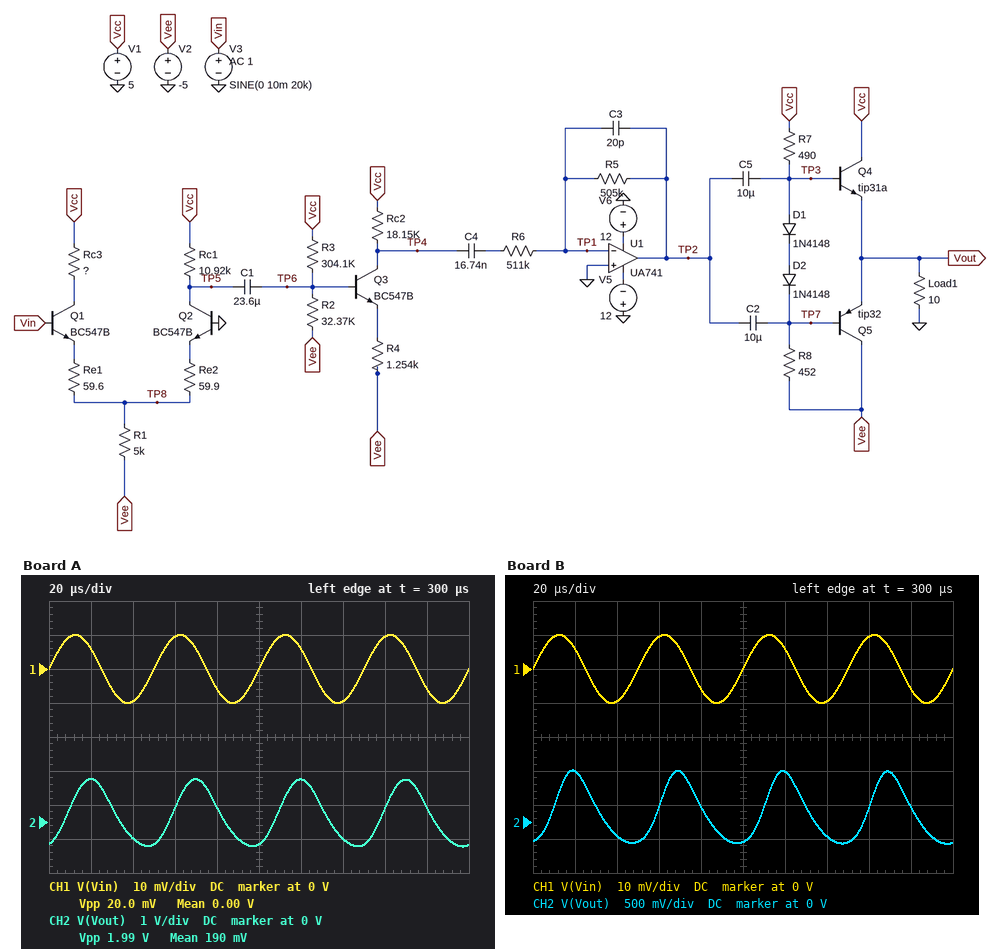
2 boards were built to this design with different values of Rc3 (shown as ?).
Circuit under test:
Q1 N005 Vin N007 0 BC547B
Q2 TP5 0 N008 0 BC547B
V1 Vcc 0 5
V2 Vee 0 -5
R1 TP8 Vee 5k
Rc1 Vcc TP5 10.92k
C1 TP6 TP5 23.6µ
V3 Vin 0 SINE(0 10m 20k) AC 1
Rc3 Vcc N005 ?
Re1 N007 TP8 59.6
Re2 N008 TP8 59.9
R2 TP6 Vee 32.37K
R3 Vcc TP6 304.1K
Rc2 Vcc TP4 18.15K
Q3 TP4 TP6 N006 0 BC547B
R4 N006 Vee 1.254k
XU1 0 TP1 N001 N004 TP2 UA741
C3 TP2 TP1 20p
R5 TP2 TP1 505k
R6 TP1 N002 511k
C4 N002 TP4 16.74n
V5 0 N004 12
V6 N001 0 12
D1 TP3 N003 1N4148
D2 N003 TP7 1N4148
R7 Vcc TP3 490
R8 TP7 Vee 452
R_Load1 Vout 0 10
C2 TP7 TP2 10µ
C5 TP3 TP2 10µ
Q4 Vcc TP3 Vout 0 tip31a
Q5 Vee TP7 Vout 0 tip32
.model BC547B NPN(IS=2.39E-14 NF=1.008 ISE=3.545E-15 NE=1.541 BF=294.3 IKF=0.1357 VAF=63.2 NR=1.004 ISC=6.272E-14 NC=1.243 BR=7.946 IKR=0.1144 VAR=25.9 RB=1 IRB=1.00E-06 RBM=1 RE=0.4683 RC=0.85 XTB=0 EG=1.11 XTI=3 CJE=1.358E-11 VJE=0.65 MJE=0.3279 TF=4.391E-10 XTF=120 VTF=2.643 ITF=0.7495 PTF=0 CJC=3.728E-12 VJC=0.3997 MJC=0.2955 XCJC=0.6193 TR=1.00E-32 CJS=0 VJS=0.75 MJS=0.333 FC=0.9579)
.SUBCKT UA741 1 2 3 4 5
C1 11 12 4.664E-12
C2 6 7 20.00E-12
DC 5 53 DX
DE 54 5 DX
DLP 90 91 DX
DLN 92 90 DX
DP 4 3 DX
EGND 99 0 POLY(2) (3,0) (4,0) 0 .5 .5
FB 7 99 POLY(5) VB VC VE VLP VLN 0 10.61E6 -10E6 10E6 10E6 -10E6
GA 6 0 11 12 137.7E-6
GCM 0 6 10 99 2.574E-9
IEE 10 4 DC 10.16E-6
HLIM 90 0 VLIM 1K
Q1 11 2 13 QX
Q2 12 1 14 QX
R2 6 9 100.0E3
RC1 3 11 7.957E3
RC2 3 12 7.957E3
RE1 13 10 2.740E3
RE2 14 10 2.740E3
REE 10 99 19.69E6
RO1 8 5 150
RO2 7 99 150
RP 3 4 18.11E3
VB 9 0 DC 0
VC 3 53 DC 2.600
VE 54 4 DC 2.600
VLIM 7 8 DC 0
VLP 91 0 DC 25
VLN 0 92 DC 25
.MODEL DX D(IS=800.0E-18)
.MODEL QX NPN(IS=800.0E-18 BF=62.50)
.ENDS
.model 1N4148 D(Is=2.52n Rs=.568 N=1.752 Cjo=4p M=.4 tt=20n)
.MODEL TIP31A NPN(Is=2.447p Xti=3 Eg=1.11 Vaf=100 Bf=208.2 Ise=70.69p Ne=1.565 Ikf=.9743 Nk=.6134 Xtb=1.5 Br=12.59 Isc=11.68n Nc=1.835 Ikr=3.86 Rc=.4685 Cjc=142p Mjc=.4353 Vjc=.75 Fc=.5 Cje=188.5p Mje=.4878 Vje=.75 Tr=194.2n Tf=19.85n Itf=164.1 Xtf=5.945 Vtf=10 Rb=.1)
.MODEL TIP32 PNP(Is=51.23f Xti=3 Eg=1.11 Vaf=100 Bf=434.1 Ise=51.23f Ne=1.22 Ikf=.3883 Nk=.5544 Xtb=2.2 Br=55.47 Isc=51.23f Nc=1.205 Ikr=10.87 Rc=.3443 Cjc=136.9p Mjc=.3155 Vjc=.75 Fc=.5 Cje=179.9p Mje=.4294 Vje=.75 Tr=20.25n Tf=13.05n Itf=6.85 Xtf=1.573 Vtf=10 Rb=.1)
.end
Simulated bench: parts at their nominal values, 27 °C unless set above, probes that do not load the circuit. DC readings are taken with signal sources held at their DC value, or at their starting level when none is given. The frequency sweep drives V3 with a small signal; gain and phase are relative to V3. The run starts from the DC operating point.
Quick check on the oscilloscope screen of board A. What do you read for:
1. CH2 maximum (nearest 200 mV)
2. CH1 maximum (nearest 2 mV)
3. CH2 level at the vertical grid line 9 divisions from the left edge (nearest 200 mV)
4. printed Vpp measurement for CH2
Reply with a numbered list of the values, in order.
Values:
1. 1.2 V
2. 10 mV
3. 400 mV
4. 1.99 V
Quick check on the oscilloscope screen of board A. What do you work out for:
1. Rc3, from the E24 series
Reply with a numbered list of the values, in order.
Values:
1. 18 kΩ
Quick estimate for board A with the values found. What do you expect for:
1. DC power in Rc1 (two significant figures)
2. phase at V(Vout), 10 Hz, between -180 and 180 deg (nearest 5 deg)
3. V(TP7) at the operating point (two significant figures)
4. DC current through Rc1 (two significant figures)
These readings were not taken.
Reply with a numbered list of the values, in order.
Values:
1. 2.7 mW
2. 140 deg
3. -830 mV
4. 500 µA
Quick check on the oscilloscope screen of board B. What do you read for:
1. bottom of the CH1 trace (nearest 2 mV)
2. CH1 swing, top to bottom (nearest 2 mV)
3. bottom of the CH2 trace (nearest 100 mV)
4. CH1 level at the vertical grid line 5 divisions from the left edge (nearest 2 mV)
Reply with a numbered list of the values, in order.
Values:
1. -10 mV
2. 20 mV
3. -300 mV
4. 0 V
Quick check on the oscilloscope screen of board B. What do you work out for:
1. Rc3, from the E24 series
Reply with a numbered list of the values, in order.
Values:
1. 20 kΩ
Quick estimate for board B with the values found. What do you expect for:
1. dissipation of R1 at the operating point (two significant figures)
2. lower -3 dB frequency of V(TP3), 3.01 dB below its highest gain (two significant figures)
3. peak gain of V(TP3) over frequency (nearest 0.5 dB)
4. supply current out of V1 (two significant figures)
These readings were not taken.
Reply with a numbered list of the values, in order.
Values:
1. 3.8 mW
2. 48 Hz
3. 36.0 dB
4. 100 mA
